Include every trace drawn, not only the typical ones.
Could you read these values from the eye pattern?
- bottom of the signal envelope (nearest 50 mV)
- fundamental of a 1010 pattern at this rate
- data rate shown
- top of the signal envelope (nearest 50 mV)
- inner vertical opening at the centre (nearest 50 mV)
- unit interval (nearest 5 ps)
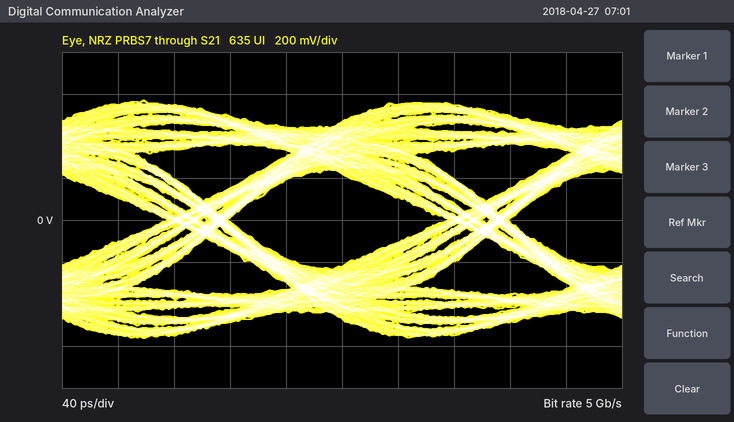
-550 mV
2.5 GHz
5 Gb/s
550 mV
450 mV
200 ps
